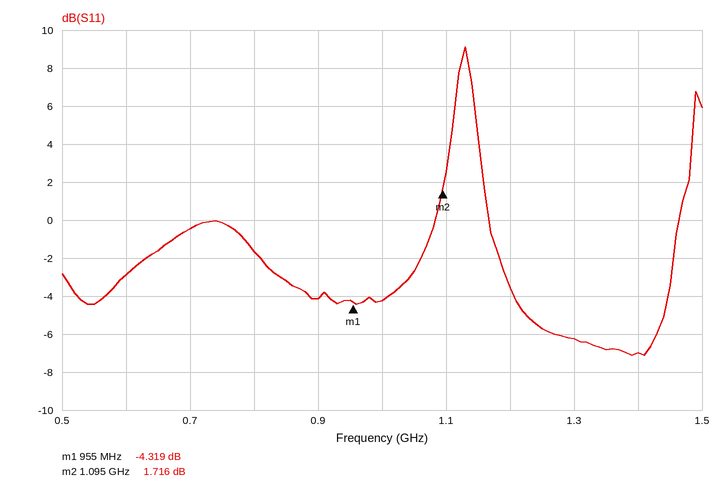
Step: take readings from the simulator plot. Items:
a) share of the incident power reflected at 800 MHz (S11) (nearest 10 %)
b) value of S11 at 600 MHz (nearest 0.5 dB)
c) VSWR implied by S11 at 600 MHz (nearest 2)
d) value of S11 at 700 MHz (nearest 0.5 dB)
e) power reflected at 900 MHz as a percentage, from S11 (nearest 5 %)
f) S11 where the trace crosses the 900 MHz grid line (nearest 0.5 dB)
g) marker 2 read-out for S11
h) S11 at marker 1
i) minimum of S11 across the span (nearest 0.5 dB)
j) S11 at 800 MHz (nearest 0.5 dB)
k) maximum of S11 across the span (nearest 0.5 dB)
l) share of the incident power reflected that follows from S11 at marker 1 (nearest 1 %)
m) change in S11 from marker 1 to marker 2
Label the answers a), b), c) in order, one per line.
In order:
a) 70 %
b) -3.0 dB
c) 6
d) -0.5 dB
e) 40 %
f) -4.0 dB
g) 1.716 dB
h) -4.319 dB
i) -7.0 dB
j) -1.5 dB
k) 9.0 dB
l) 37 %
m) 6.035 dB
